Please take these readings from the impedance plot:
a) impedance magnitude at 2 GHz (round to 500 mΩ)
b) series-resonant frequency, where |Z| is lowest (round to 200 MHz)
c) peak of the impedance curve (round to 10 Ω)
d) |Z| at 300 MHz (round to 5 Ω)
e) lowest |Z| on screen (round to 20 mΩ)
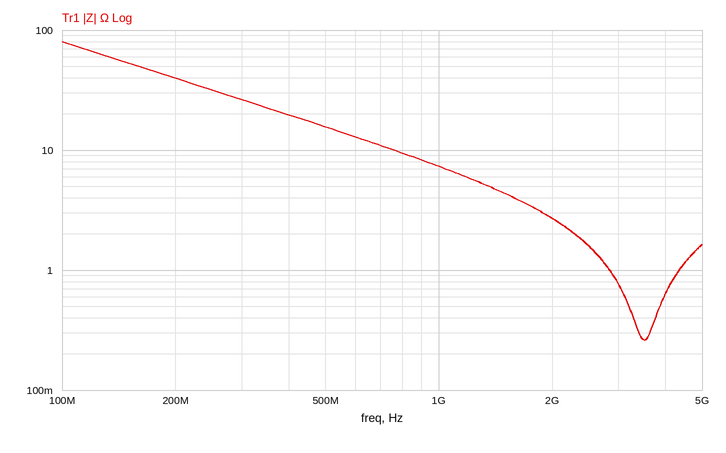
2.5 Ω
3.6 GHz
80 Ω
25 Ω
260 mΩ
